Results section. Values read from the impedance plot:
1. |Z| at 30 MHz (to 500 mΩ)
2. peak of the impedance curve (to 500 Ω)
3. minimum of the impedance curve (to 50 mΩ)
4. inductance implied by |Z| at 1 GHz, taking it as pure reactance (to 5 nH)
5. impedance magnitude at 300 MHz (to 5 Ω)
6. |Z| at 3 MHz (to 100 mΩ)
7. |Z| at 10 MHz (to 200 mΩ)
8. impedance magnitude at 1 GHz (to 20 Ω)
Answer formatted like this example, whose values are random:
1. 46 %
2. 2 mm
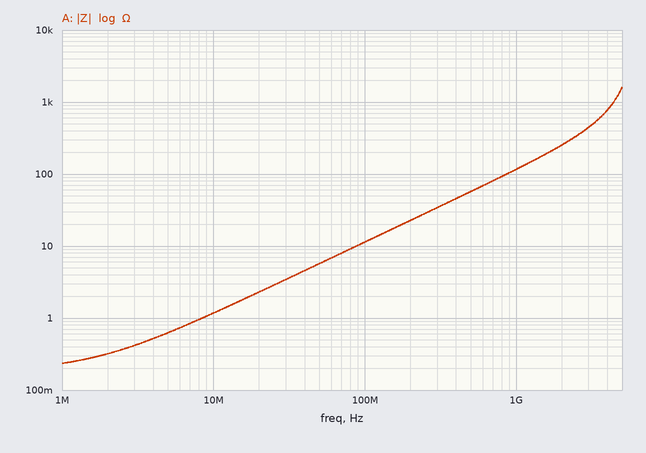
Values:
1. 3.5 Ω
2. 1.5 kΩ
3. 250 mΩ
4. 20 nH
5. 35 Ω
6. 400 mΩ
7. 1.2 Ω
8. 120 Ω
